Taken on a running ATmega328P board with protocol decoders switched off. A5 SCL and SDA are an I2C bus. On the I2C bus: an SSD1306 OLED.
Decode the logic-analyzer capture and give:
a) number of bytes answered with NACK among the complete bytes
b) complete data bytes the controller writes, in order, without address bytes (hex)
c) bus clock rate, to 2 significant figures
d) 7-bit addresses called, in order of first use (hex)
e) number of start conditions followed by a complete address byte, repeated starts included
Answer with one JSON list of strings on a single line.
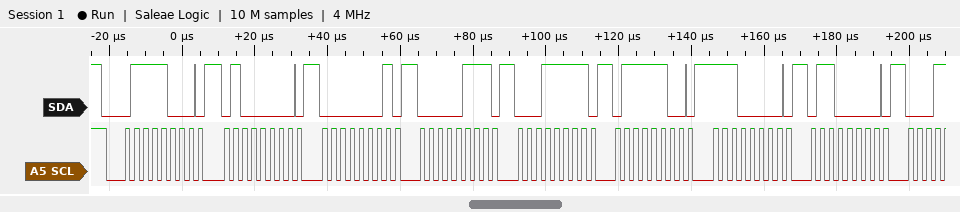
["0", "40 01 07 1F 7C E0 60", "400 kHz", "0x3C", "1"]
